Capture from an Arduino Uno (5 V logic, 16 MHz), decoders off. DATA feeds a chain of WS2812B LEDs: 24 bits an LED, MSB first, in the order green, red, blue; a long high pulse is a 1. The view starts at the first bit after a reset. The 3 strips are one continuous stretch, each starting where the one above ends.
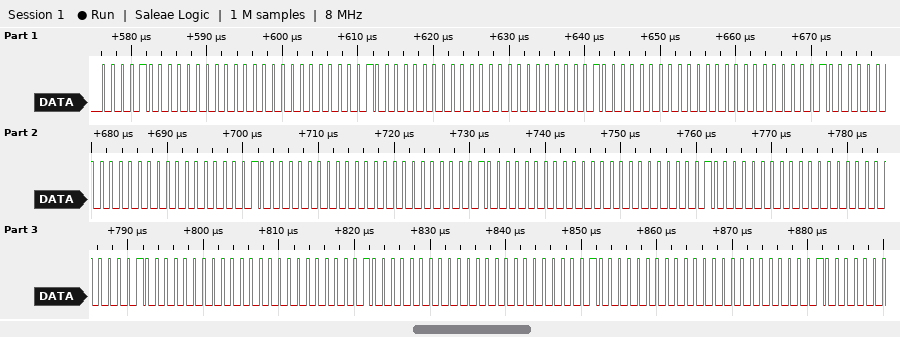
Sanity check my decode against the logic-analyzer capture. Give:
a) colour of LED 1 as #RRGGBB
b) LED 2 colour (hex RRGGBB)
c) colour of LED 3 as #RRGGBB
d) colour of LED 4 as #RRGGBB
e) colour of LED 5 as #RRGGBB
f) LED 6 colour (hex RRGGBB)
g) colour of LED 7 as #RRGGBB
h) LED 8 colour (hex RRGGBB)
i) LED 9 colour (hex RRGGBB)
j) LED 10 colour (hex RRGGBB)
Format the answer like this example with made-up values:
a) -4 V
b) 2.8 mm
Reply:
a) #000800
b) #000800
c) #000800
d) #000800
e) #000800
f) #000800
g) #000800
h) #000800
i) #000800
j) #000800
